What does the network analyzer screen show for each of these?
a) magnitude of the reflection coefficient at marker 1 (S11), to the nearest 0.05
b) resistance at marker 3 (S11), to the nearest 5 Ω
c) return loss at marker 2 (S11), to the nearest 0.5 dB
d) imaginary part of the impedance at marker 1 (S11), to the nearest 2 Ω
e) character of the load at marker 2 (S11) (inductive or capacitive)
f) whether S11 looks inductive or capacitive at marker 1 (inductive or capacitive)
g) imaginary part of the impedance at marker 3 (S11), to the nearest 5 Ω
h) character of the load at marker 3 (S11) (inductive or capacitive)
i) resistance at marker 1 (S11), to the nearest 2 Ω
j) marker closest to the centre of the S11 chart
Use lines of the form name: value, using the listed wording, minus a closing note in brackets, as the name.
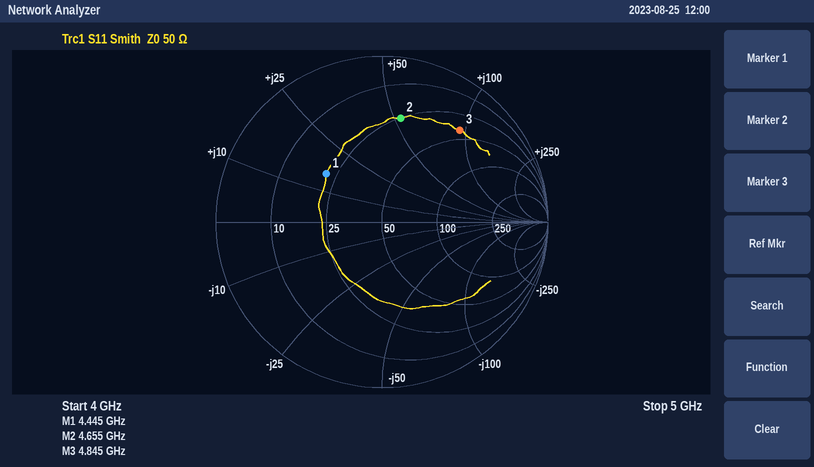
magnitude of the reflection coefficient at marker 1 (S11), to the nearest 0.05: 0.45
resistance at marker 3 (S11), to the nearest 5 Ω: 40 Ω
return loss at marker 2 (S11), to the nearest 0.5 dB: 4.0 dB
imaginary part of the impedance at marker 1 (S11), to the nearest 2 Ω: +16 Ω
character of the load at marker 2 (S11): inductive
whether S11 looks inductive or capacitive at marker 1: inductive
imaginary part of the impedance at marker 3 (S11), to the nearest 5 Ω: +95 Ω
character of the load at marker 3 (S11): inductive
resistance at marker 1 (S11), to the nearest 2 Ω: 22 Ω
marker closest to the centre of the S11 chart: marker 1
